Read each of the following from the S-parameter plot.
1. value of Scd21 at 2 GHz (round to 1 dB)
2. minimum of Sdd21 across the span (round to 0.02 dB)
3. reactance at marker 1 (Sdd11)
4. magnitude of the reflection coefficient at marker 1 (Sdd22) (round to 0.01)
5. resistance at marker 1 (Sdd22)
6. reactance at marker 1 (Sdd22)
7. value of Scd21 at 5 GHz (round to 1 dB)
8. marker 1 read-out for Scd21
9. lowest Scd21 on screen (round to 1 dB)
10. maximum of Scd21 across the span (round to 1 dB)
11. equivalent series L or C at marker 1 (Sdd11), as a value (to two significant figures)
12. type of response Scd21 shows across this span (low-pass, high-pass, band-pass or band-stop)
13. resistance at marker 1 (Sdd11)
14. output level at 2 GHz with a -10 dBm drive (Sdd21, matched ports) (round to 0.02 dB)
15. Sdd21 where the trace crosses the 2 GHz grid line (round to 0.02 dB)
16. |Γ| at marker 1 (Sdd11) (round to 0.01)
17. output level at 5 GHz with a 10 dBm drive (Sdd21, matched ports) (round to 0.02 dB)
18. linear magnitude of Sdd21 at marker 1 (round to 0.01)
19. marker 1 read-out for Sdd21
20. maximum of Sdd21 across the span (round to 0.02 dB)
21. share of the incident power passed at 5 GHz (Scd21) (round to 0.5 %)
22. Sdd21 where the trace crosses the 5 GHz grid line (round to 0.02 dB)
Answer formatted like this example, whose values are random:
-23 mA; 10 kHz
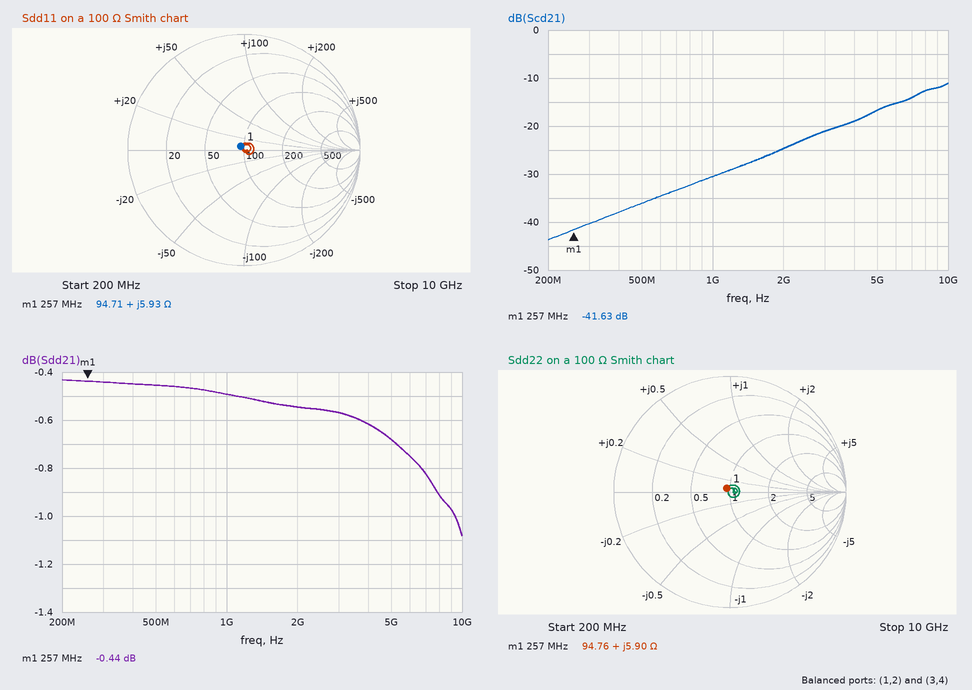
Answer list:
-25 dB; -1.08 dB; +5.93 Ω; 0.04; 94.76 Ω; +5.90 Ω; -17 dB; -41.63 dB; -44 dB; -11 dB; 3.7 nH; high-pass; 94.71 Ω; -10.54 dBm; -0.54 dB; 0.04; 9.32 dBm; 0.95; -0.44 dB; -0.44 dB; 2.0 %; -0.68 dB
